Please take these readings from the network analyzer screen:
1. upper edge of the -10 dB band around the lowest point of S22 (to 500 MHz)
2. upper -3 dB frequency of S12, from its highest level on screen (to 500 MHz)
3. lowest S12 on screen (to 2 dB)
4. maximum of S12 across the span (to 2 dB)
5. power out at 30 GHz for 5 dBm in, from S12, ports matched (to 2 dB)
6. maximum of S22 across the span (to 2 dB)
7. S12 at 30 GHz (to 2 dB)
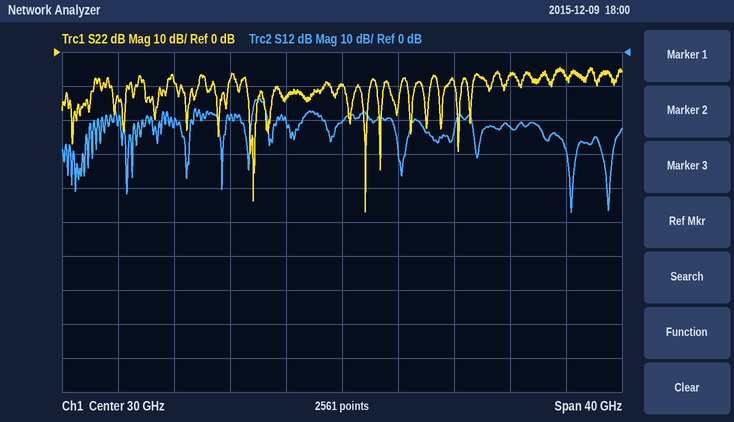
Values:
32.0 GHz
24.5 GHz
-48 dB
-14 dB
-16 dBm
-4 dB
-20 dB
